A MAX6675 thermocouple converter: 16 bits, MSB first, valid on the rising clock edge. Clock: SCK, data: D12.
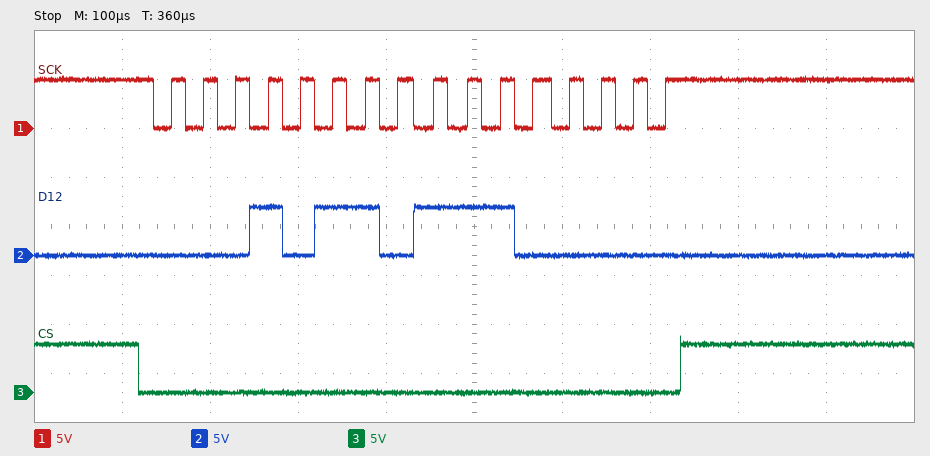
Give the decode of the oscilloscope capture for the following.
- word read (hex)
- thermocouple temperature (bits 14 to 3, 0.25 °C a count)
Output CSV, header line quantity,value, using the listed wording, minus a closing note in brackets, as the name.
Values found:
quantity,value
word read,0x16E0
thermocouple temperature,183.00 °C
